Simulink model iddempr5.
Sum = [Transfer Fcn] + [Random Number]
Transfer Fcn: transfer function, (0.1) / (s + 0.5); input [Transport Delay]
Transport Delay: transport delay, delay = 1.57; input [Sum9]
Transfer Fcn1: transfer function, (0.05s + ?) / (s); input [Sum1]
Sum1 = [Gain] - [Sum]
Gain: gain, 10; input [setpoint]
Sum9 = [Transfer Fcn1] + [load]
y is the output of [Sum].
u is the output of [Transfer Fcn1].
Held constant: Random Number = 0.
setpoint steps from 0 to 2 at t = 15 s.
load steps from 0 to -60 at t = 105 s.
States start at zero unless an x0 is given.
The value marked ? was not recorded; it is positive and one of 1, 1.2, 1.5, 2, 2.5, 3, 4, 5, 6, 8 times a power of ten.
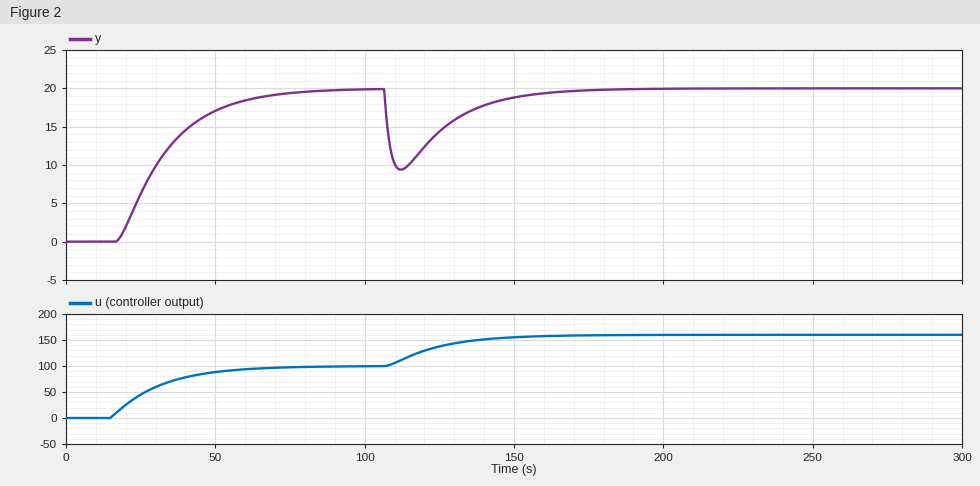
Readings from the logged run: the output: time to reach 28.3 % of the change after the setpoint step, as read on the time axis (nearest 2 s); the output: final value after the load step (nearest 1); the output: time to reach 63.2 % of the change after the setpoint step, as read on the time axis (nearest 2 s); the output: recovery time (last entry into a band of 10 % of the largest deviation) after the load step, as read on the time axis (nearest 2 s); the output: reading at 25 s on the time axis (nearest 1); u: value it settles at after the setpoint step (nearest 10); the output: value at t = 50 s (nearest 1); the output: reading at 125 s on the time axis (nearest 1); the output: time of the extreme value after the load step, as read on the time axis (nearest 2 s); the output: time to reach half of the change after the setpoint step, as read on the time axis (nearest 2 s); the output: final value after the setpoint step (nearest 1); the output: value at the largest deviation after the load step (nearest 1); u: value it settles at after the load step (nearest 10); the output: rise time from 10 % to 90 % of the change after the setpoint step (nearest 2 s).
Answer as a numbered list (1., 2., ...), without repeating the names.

1. 24 s
2. 20
3. 36 s
4. 152 s
5. 6
6. 100
7. 17
8. 14
9. 112 s
10. 30 s
11. 20
12. 9
13. 160
14. 36 s
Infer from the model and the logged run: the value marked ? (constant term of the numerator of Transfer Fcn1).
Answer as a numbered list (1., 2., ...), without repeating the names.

1. 0.25
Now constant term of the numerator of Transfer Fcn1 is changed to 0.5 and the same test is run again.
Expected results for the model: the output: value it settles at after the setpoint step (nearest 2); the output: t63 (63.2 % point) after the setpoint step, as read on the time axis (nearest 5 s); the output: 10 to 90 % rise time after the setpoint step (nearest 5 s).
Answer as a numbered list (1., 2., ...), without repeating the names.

1. 20
2. 25 s
3. 15 s
